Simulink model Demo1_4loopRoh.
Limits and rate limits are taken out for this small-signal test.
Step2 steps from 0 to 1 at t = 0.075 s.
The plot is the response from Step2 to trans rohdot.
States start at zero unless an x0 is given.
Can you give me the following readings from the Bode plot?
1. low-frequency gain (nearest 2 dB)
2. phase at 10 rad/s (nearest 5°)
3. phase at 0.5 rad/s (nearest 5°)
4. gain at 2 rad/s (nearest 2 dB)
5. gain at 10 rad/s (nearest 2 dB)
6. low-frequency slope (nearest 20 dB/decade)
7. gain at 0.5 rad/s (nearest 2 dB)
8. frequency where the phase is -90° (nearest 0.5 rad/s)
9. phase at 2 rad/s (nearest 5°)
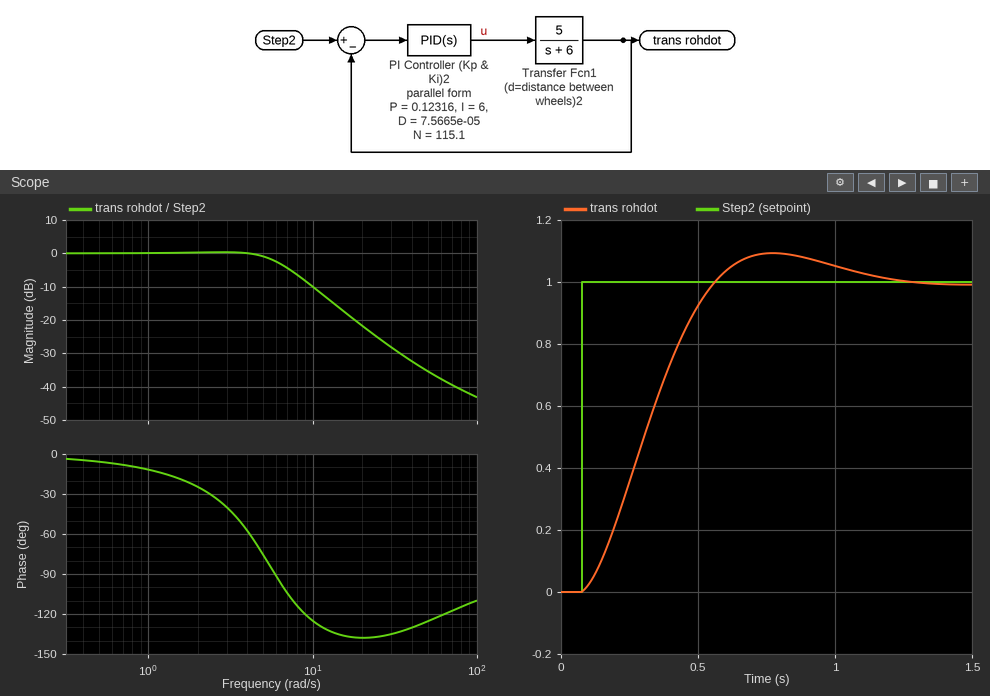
0 dB
-125°
-5°
0 dB
-10 dB
0 dB/decade
0 dB
6.0 rad/s
-25°
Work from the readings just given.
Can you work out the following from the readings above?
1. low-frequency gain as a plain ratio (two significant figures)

1.0
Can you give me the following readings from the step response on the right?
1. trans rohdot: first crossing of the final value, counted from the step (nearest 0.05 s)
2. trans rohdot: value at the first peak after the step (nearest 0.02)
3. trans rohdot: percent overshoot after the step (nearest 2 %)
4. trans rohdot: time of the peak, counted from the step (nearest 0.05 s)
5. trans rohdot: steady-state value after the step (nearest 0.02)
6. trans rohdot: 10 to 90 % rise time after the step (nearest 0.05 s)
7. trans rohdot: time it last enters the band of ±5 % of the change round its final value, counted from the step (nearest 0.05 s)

0.50 s
1.10
10 %
0.70 s
1.00
0.35 s
0.95 s
